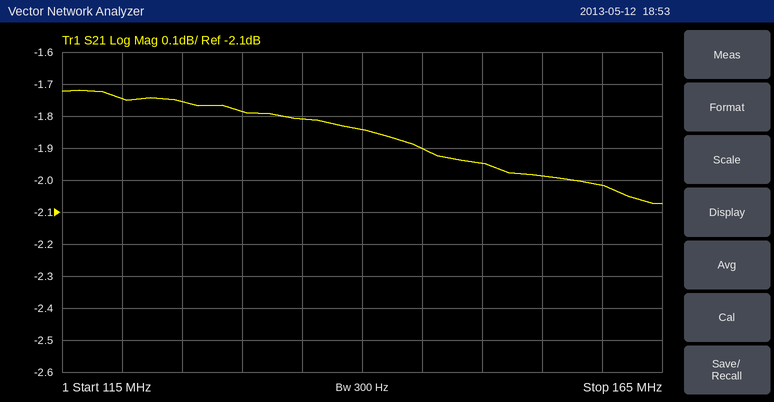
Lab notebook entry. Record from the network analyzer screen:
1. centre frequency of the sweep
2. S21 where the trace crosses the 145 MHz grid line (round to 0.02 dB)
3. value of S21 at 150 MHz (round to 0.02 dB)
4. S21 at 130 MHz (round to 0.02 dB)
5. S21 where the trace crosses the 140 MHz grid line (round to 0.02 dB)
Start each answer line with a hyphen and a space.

- 140 MHz
- -1.90 dB
- -1.94 dB
- -1.78 dB
- -1.84 dB
